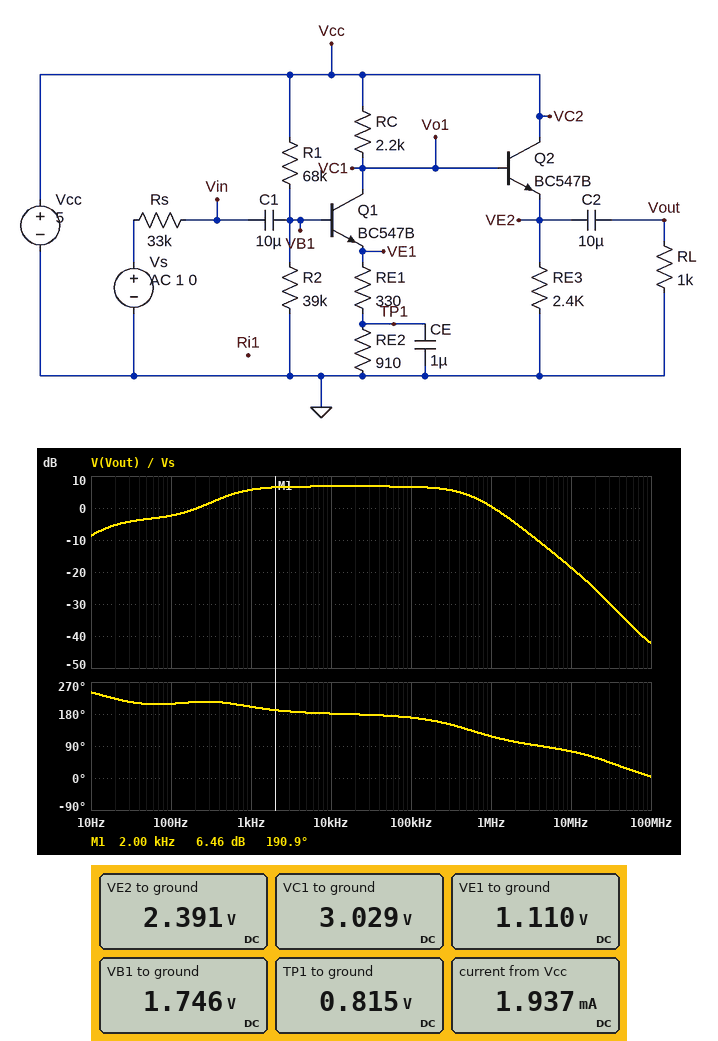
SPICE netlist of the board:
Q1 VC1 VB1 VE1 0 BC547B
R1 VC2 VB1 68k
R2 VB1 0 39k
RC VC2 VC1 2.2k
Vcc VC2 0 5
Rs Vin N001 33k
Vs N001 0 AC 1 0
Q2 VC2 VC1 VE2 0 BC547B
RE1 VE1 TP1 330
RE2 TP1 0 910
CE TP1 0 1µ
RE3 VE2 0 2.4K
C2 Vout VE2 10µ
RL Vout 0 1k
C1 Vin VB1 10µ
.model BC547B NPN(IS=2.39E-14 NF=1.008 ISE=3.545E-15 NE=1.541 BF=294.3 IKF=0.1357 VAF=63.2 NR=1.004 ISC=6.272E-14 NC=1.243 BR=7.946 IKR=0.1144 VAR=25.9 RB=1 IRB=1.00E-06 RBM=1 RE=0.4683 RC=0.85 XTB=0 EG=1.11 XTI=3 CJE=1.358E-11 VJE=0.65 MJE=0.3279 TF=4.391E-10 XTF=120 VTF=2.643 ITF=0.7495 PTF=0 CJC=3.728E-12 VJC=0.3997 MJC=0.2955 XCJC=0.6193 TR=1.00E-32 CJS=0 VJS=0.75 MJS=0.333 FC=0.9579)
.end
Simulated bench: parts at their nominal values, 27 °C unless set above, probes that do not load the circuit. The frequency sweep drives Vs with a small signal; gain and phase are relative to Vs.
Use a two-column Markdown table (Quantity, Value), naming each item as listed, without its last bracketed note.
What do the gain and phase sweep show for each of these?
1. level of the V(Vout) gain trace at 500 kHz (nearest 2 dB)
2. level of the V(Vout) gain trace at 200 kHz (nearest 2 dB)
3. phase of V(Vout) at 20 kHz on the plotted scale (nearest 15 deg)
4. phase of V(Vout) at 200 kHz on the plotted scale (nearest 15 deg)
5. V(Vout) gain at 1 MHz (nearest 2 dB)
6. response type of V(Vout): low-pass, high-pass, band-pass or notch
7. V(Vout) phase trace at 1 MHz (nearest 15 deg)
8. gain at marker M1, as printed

| Quantity | Value |
|---|---|
| level of the V(Vout) gain trace at 500 kHz | 4 dB |
| level of the V(Vout) gain trace at 200 kHz | 6 dB |
| phase of V(Vout) at 20 kHz on the plotted scale | 180 deg |
| phase of V(Vout) at 200 kHz on the plotted scale | 165 deg |
| V(Vout) gain at 1 MHz | 0 dB |
| response type of V(Vout): low-pass, high-pass, band-pass or notch | band-pass |
| V(Vout) phase trace at 1 MHz | 120 deg |
| gain at marker M1, as printed | 6.46 dB |
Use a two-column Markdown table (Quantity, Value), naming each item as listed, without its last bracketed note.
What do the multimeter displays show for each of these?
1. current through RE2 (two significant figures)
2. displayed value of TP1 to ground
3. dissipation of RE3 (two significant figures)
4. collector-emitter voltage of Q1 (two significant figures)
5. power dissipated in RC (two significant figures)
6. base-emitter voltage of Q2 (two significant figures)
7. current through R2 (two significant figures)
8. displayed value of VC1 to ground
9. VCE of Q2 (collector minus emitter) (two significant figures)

| Quantity | Value |
|---|---|
| current through RE2 | 900 µA |
| displayed value of TP1 to ground | 0.815 V |
| dissipation of RE3 | 2.4 mW |
| collector-emitter voltage of Q1 | 1.9 V |
| power dissipated in RC | 1.8 mW |
| base-emitter voltage of Q2 | 640 mV |
| current through R2 | 45 µA |
| displayed value of VC1 to ground | 3.029 V |
| VCE of Q2 (collector minus emitter) | 2.6 V |
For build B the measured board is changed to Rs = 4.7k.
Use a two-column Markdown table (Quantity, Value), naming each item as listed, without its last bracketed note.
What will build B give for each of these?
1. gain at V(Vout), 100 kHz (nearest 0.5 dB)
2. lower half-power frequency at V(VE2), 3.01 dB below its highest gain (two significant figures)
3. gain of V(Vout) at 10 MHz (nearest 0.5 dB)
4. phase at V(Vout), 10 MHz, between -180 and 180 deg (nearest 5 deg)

| Quantity | Value |
|---|---|
| gain at V(Vout), 100 kHz | 13.5 dB |
| lower half-power frequency at V(VE2), 3.01 dB below its highest gain | 550 Hz |
| gain of V(Vout) at 10 MHz | -2.5 dB |
| phase at V(Vout), 10 MHz, between -180 and 180 deg | 80 deg |
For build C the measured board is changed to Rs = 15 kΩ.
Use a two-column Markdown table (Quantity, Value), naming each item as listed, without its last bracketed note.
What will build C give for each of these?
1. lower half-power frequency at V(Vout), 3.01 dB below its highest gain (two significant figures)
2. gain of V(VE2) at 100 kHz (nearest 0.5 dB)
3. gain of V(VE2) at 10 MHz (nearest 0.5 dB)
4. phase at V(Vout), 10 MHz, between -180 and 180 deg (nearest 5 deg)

| Quantity | Value |
|---|---|
| lower half-power frequency at V(Vout), 3.01 dB below its highest gain | 520 Hz |
| gain of V(VE2) at 100 kHz | 10.5 dB |
| gain of V(VE2) at 10 MHz | -12.0 dB |
| phase at V(Vout), 10 MHz, between -180 and 180 deg | 75 deg |
